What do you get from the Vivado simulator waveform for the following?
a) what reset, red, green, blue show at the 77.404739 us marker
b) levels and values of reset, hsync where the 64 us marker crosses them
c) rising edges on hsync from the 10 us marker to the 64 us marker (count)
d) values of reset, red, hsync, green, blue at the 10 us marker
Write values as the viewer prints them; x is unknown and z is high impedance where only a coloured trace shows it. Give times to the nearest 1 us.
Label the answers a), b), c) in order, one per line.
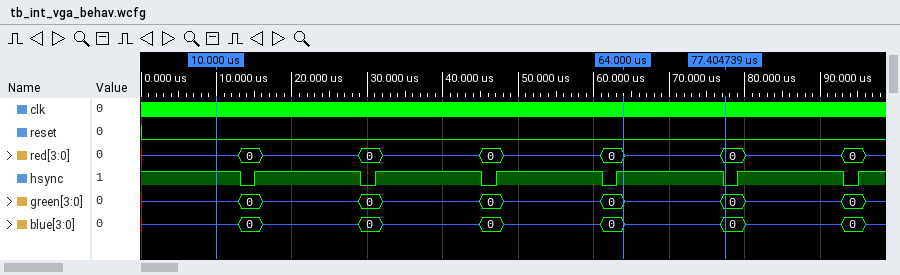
a) reset=0, red=0, green=0, blue=0
b) reset=0, hsync=1
c) 4
d) reset=0, red=z, hsync=1, green=z, blue=z
